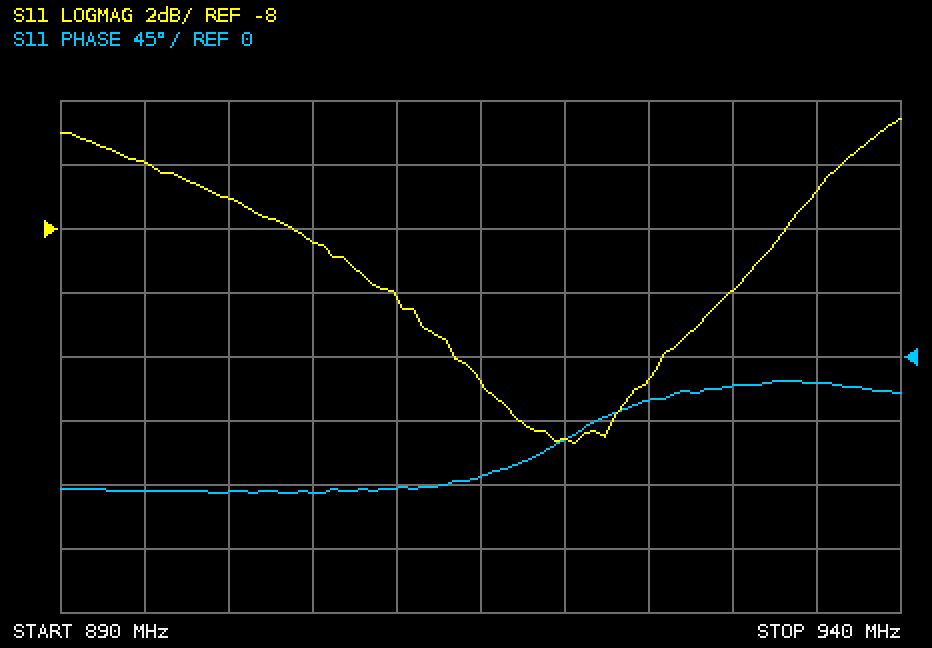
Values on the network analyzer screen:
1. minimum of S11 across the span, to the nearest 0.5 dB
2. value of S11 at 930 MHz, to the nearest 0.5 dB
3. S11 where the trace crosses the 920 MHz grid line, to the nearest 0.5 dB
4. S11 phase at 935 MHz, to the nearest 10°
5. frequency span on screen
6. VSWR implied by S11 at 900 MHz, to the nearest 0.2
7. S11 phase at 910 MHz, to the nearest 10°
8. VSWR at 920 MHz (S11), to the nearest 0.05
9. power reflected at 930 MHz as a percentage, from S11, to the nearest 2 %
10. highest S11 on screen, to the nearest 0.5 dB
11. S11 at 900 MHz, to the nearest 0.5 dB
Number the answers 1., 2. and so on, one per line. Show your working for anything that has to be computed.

1. -14.5 dB
2. -10.0 dB
3. -14.5 dB
4. -20°
5. 50 MHz
6. |Γ| = 10^(-7/20) = 0.4467; VSWR = (1 + 0.4467)/(1 − 0.4467) ≈ 2.6
7. -90°
8. |Γ| = 10^(-14.5/20) = 0.1884; VSWR = (1 + 0.1884)/(1 − 0.1884) ≈ 1.46, so 1.45 to the nearest 0.05
9. 10^(-10/10) ≈ 10 %
10. -4.5 dB
11. -7.0 dB
